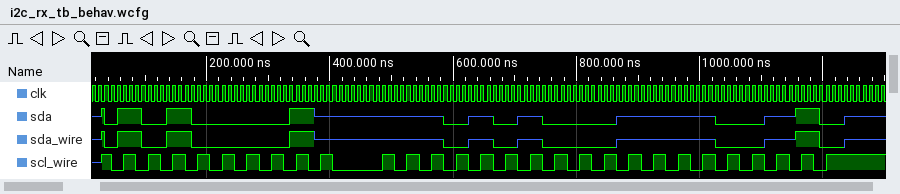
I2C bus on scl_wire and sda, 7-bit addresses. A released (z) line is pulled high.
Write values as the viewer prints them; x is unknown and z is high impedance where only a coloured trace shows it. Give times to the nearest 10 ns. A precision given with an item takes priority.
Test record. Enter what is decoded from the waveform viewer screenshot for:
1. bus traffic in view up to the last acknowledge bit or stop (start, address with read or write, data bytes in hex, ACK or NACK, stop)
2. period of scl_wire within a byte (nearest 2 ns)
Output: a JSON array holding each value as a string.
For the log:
["start, address 50 read NACK, EA ACK, 79 NACK, stop", "40 ns"]
